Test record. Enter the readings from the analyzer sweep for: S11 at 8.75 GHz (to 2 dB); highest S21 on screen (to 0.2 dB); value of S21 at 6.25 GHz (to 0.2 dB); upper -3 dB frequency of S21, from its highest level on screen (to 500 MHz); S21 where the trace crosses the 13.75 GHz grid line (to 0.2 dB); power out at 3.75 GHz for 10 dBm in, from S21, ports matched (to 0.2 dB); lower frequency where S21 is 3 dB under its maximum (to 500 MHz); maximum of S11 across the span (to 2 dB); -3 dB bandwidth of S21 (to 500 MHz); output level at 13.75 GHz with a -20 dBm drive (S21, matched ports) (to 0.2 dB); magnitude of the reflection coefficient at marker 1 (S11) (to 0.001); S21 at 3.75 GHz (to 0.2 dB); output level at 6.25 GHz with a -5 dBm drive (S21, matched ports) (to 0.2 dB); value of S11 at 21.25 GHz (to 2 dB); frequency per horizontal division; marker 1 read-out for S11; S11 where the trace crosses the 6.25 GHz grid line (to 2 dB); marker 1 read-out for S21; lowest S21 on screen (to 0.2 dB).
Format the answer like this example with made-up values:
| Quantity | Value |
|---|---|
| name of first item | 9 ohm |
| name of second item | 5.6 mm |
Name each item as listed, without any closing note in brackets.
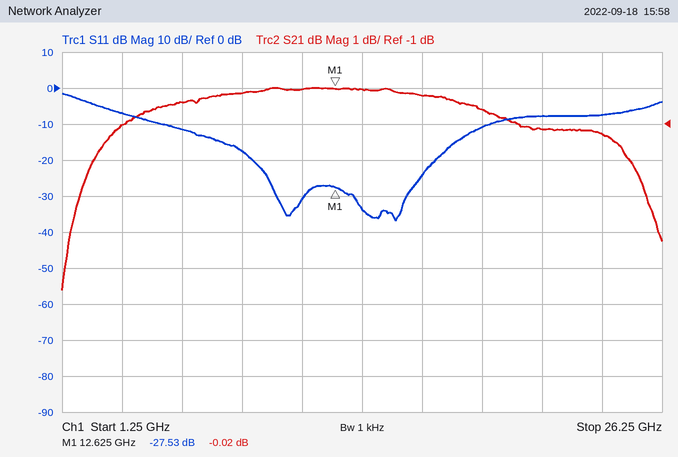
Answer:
| Quantity | Value |
|---|---|
| S11 at 8.75 GHz | -18 dB |
| highest S21 on screen | 0.0 dB |
| value of S21 at 6.25 GHz | -0.4 dB |
| upper -3 dB frequency of S21, from its highest level on screen | 25.5 GHz |
| S21 where the trace crosses the 13.75 GHz grid line | 0.0 dB |
| power out at 3.75 GHz for 10 dBm in, from S21, ports matched | 9.0 dBm |
| lower frequency where S21 is 3 dB under its maximum | 2.0 GHz |
| maximum of S11 across the span | -2 dB |
| -3 dB bandwidth of S21 | 23.5 GHz |
| output level at 13.75 GHz with a -20 dBm drive (S21, matched ports) | -20.0 dBm |
| magnitude of the reflection coefficient at marker 1 (S11) | 0.042 |
| S21 at 3.75 GHz | -1.0 dB |
| output level at 6.25 GHz with a -5 dBm drive (S21, matched ports) | -5.4 dBm |
| value of S11 at 21.25 GHz | -8 dB |
| frequency per horizontal division | 2.5 GHz |
| marker 1 read-out for S11 | -27.53 dB |
| S11 where the trace crosses the 6.25 GHz grid line | -12 dB |
| marker 1 read-out for S21 | -0.02 dB |
| lowest S21 on screen | -5.6 dB |
